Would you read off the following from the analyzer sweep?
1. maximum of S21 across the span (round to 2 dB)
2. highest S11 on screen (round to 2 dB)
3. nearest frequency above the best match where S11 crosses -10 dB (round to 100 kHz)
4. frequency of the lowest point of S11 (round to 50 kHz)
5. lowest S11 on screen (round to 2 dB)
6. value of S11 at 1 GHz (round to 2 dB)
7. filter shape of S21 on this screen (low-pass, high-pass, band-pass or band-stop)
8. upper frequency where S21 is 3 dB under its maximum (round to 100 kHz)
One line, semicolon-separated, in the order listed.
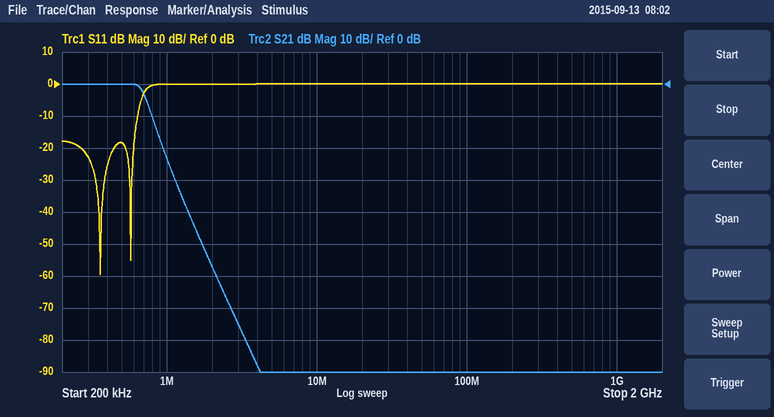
0 dB; 0 dB; 600 kHz; 350 kHz; -60 dB; 0 dB; low-pass; 700 kHz
